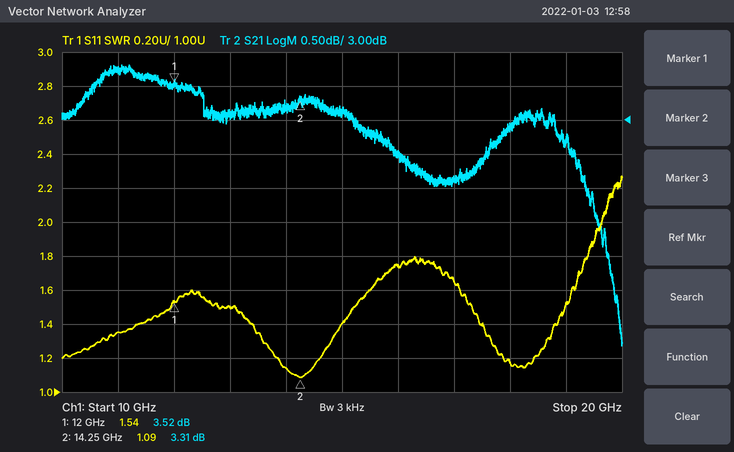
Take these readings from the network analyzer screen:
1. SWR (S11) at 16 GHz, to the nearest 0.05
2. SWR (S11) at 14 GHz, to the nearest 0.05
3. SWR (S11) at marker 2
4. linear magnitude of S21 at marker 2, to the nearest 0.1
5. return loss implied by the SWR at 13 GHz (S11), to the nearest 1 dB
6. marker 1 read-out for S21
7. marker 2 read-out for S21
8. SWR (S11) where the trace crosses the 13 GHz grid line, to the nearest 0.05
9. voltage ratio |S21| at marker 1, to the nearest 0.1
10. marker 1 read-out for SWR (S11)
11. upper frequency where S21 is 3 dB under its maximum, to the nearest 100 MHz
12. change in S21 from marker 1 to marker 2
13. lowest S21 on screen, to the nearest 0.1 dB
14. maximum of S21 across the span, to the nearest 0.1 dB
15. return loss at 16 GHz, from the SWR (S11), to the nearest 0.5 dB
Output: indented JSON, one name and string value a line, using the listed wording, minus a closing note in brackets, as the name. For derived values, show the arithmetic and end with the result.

{
  "SWR (S11) at 16 GHz, to the nearest 0.05": "1.75",
  "SWR (S11) at 14 GHz, to the nearest 0.05": "1.15",
  "SWR (S11) at marker 2": "1.09",
  "linear magnitude of S21 at marker 2, to the nearest 0.1": "10^(3.31/20) ≈ 1.5",
  "return loss implied by the SWR at 13 GHz (S11), to the nearest 1 dB": "−20 log10((1.5 − 1)/(1.5 + 1)) ≈ 14 dB",
  "marker 1 read-out for S21": "3.52 dB",
  "marker 2 read-out for S21": "3.31 dB",
  "SWR (S11) where the trace crosses the 13 GHz grid line, to the nearest 0.05": "1.50",
  "voltage ratio |S21| at marker 1, to the nearest 0.1": "10^(3.52/20) ≈ 1.5",
  "marker 1 read-out for SWR": "1.54",
  "upper frequency where S21 is 3 dB under its maximum, to the nearest 100 MHz": "19.8 GHz",
  "change in S21 from marker 1 to marker 2": "3.31 − (3.52) = -0.21 dB",
  "lowest S21 on screen, to the nearest 0.1 dB": "-0.3 dB",
  "maximum of S21 across the span, to the nearest 0.1 dB": "3.8 dB",
  "return loss at 16 GHz, from the SWR (S11), to the nearest 0.5 dB": "−20 log10((1.75 − 1)/(1.75 + 1)) ≈ 11.3 dB, so 11.5 dB to the nearest 0.5 dB"
}
